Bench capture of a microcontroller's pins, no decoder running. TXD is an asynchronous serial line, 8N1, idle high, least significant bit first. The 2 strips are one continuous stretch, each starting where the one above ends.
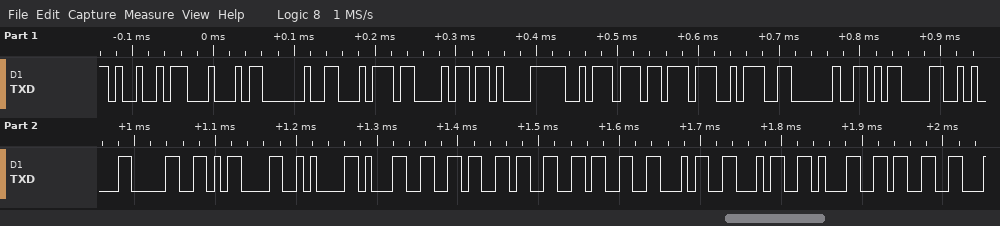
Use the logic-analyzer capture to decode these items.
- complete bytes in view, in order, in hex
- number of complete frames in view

0x49 0x44 0x20 0x74 0x68 0xE1 0xBA 0xBB 0x3A 0x20 0x0D 0x0A 0x30 0x0D 0x0A 0x31 0x36 0x33 0x33 0x34 0x34 0x31 0x33
23
